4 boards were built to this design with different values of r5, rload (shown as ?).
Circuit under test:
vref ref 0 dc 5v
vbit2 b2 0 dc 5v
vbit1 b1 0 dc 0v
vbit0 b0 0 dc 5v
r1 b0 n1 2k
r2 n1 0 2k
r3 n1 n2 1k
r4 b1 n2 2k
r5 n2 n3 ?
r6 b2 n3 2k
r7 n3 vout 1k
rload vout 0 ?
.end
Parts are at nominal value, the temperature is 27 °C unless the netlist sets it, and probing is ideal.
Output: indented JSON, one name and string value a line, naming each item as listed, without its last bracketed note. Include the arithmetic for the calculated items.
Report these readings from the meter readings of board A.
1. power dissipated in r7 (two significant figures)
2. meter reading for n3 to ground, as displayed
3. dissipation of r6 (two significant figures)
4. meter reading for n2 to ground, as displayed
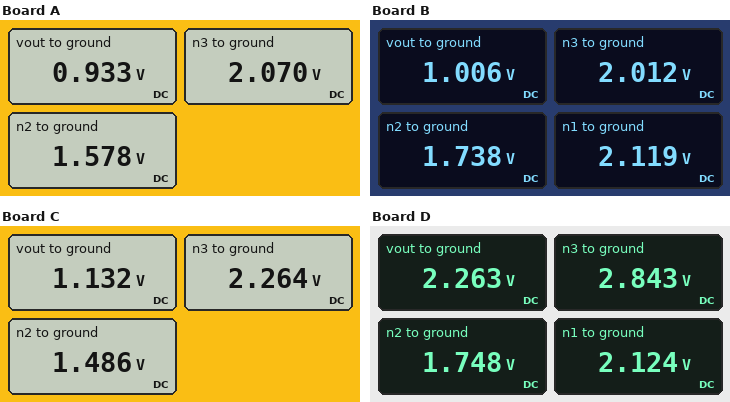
{
  "power dissipated in r7": "(2.07 V - 933 mV)^2 / 1 kΩ = 1.3 mW",
  "meter reading for n3 to ground, as displayed": "2.070 V",
  "dissipation of r6": "(5 V - 2.07 V)^2 / 2 kΩ = 4.3 mW",
  "meter reading for n2 to ground, as displayed": "1.578 V"
}
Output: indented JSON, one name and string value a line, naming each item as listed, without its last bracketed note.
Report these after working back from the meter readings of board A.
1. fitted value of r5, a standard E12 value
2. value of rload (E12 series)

{
  "fitted value of r5, a standard E12 value": "1.5 kΩ",
  "value of rload": "820 Ω"
}
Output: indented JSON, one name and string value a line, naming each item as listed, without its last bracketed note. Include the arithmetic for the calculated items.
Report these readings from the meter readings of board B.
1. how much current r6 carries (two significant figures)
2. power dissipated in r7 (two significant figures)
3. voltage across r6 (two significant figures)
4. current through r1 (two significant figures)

{
  "how much current r6 carries": "(5 V - 2.012 V) / 2 kΩ = 1.5 mA",
  "power dissipated in r7": "(2.012 V - 1.006 V)^2 / 1 kΩ = 1.0 mW",
  "voltage across r6": "5 V - 2.012 V = 3.0 V",
  "current through r1": "(5 V - 2.119 V) / 2 kΩ = 1.4 mA"
}
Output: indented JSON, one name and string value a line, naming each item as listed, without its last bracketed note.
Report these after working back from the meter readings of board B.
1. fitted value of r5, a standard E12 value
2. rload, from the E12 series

{
  "fitted value of r5, a standard E12 value": "560 Ω",
  "rload, from the E12 series": "1 kΩ"
}
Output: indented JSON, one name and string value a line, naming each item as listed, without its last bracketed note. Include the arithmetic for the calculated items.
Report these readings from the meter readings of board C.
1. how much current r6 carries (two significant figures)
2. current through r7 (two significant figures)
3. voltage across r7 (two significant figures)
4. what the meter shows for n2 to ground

{
  "how much current r6 carries": "(5 V - 2.264 V) / 2 kΩ = 1.4 mA",
  "current through r7": "(2.264 V - 1.132 V) / 1 kΩ = 1.1 mA",
  "voltage across r7": "2.264 V - 1.132 V = 1.1 V",
  "what the meter shows for n2 to ground": "1.486 V"
}
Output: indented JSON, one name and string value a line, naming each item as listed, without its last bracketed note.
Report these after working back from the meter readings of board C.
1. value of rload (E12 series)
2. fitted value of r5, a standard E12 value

{
  "value of rload": "1 kΩ",
  "fitted value of r5, a standard E12 value": "3.3 kΩ"
}
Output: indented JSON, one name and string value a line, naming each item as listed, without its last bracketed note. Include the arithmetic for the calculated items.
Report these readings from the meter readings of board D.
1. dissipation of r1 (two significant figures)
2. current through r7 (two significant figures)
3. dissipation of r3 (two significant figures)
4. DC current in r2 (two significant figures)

{
  "dissipation of r1": "(5 V - 2.124 V)^2 / 2 kΩ = 4.1 mW",
  "current through r7": "(2.843 V - 2.263 V) / 1 kΩ = 580 µA",
  "dissipation of r3": "(2.124 V - 1.748 V)^2 / 1 kΩ = 140 µW",
  "DC current in r2": "(2.124 V) / 2 kΩ = 1.1 mA"
}
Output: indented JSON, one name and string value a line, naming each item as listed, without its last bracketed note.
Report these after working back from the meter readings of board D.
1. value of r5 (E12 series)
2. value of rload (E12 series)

{
  "value of r5": "2.2 kΩ",
  "value of rload": "3.9 kΩ"
}
